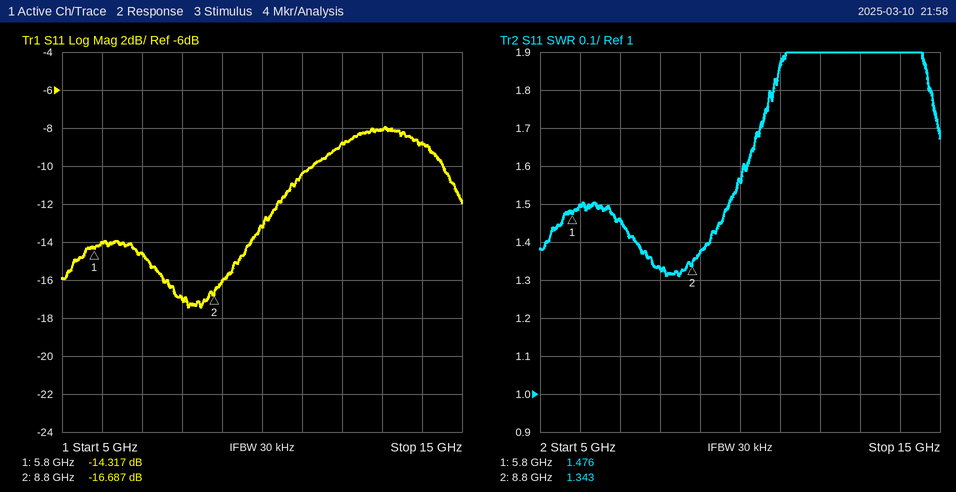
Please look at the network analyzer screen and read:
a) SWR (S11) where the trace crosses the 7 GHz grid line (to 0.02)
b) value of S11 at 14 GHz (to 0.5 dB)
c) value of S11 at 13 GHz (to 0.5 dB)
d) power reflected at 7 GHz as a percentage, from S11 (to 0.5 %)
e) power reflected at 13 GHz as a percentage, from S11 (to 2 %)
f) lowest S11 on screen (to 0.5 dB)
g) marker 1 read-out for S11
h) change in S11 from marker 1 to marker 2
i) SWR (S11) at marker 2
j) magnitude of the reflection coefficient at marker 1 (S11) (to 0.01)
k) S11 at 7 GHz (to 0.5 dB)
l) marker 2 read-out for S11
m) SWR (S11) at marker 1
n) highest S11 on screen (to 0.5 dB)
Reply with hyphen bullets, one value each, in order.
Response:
- 1.46
- -9.0 dB
- -8.0 dB
- 3.5 %
- 16 %
- -17.5 dB
- -14.317 dB
- -2.370 dB
- 1.343
- 0.19
- -14.5 dB
- -16.687 dB
- 1.476
- -8.0 dB
